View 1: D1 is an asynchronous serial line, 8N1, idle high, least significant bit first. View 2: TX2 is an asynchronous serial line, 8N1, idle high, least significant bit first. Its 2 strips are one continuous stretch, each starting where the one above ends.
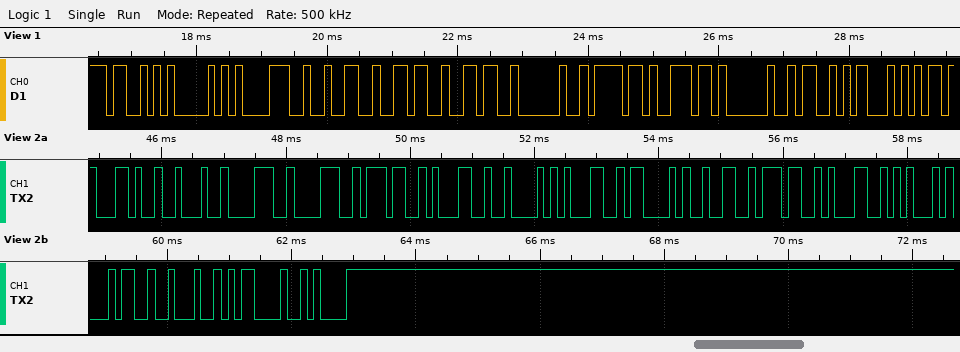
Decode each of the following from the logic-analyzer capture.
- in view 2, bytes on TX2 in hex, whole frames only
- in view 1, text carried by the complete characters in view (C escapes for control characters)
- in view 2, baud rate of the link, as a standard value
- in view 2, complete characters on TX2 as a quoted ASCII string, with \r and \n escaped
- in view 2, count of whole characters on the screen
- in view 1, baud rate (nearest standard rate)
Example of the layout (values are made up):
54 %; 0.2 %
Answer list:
2C 22 38 38 37 31 42 31 43 32 37 31 45 34 22 0D 0A; "SP8266 on ST"; 9600 baud; ",\"8871B1C271E4\"\r\n"; 17; 9600 baud
